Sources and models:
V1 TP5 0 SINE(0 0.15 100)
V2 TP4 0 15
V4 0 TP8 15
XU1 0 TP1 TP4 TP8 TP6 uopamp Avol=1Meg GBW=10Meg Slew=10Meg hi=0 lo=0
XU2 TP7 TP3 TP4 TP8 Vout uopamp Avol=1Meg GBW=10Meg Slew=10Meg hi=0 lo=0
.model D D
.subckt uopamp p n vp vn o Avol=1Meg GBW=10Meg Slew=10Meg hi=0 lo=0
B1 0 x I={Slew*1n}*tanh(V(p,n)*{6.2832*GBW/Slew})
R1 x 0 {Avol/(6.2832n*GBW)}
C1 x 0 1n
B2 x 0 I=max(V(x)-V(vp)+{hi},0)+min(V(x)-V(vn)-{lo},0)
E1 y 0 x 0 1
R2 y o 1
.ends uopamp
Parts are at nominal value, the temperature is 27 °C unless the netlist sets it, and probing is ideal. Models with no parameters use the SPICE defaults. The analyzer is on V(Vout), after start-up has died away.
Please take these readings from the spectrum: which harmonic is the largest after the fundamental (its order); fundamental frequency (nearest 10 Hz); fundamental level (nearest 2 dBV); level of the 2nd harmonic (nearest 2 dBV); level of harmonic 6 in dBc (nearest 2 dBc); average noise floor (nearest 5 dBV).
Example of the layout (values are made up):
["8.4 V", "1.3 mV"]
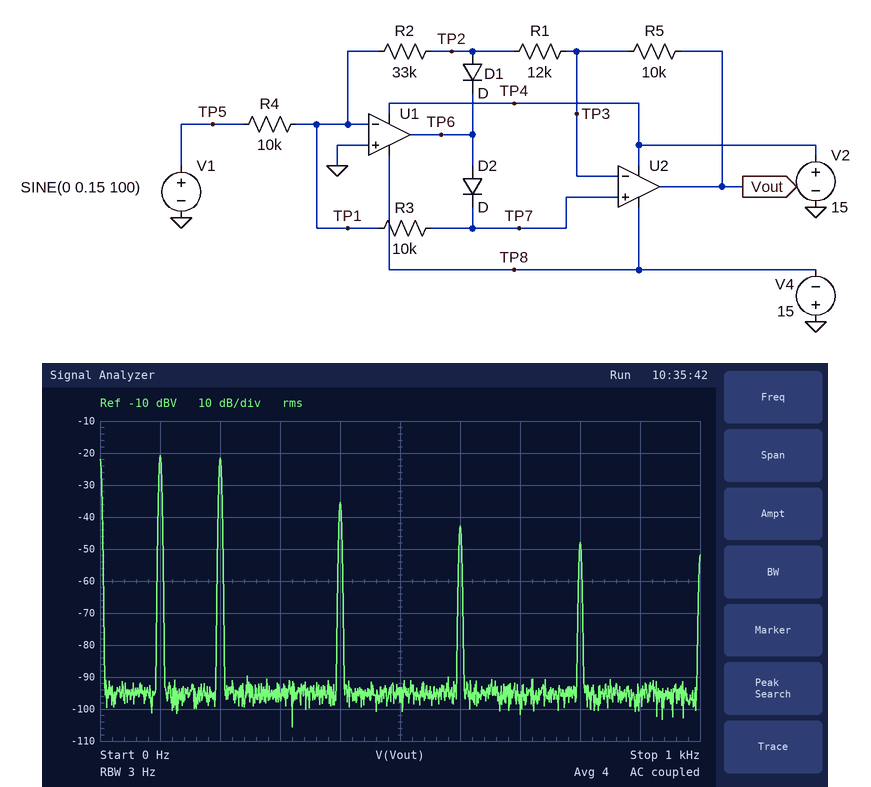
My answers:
["2", "100 Hz", "-20 dBV", "-22 dBV", "-22 dBc", "-95 dBV"]
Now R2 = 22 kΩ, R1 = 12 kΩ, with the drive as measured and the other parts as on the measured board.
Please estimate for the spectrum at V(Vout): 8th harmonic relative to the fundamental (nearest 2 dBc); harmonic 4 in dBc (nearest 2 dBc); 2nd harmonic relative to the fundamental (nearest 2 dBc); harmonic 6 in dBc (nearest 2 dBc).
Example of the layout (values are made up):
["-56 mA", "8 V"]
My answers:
["-24 dBc", "-10 dBc", "4 dBc", "-18 dBc"]
